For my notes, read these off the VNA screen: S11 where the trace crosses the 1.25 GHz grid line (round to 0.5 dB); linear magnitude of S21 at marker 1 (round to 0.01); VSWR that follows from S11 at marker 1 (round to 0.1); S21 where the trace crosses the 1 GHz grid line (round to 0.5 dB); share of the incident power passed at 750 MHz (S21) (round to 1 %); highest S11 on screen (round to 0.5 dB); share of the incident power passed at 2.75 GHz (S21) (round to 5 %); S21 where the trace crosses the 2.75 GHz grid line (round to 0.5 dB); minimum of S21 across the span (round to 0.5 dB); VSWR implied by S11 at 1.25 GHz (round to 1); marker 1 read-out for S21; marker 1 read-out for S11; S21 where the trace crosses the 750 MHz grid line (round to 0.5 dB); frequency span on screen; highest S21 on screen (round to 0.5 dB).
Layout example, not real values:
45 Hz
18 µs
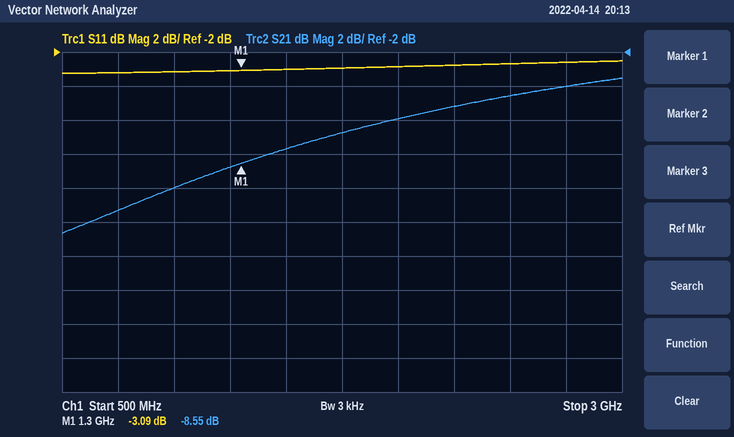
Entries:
-3.0 dB
0.37
5.7
-10.0 dB
7 %
-2.5 dB
40 %
-4.0 dB
-12.5 dB
6
-8.55 dB
-3.09 dB
-11.5 dB
2.5 GHz
-3.5 dB
